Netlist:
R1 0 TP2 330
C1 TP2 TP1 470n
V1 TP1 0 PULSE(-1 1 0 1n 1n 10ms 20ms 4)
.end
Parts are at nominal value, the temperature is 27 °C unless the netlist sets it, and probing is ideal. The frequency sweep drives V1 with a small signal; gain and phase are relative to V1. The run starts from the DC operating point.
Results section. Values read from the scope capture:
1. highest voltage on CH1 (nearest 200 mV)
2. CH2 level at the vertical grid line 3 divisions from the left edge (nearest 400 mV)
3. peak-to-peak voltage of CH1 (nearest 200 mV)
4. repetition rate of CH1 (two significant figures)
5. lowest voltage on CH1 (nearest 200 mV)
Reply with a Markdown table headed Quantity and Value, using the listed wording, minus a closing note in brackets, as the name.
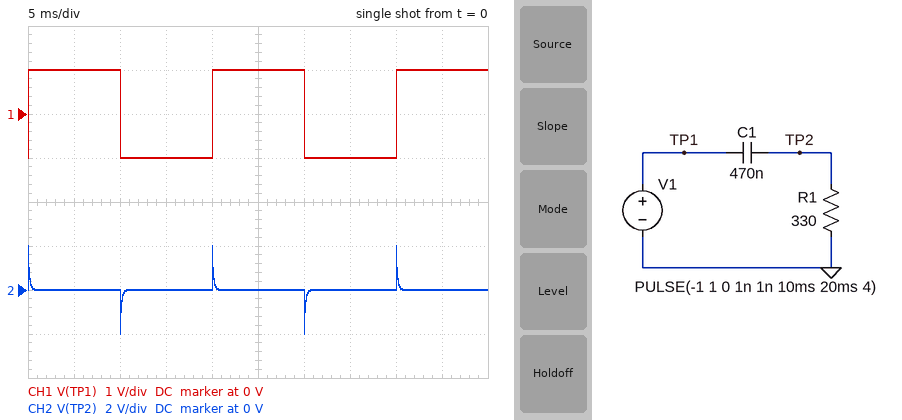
| Quantity | Value |
|---|---|
| highest voltage on CH1 | 1.0 V |
| CH2 level at the vertical grid line 3 divisions from the left edge | 0 V |
| peak-to-peak voltage of CH1 | 2.0 V |
| repetition rate of CH1 | 50 Hz |
| lowest voltage on CH1 | -1.0 V |
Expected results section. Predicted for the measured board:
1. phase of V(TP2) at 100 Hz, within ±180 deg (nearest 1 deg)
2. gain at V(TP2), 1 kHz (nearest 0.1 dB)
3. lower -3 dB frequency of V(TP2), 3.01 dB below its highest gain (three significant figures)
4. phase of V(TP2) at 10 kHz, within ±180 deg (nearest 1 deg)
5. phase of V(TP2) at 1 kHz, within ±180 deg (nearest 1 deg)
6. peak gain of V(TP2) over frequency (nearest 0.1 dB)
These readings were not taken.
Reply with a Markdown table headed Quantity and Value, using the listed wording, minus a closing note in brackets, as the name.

| Quantity | Value |
|---|---|
| phase of V(TP2) at 100 Hz, within ±180 deg | 84 deg |
| gain at V(TP2), 1 kHz | -3.1 dB |
| lower -3 dB frequency of V(TP2), 3.01 dB below its highest gain | 1.03 kHz |
| phase of V(TP2) at 10 kHz, within ±180 deg | 6 deg |
| phase of V(TP2) at 1 kHz, within ±180 deg | 46 deg |
| peak gain of V(TP2) over frequency | 0 dB |
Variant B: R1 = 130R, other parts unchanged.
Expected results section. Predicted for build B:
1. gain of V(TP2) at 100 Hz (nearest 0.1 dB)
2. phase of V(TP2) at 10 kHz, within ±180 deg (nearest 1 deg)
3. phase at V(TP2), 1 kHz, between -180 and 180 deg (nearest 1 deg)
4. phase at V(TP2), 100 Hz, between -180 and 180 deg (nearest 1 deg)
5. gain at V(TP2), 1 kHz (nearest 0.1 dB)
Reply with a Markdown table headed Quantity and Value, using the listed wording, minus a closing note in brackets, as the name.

| Quantity | Value |
|---|---|
| gain of V(TP2) at 100 Hz | -28.3 dB |
| phase of V(TP2) at 10 kHz, within ±180 deg | 15 deg |
| phase at V(TP2), 1 kHz, between -180 and 180 deg | 69 deg |
| phase at V(TP2), 100 Hz, between -180 and 180 deg | 88 deg |
| gain at V(TP2), 1 kHz | -8.9 dB |
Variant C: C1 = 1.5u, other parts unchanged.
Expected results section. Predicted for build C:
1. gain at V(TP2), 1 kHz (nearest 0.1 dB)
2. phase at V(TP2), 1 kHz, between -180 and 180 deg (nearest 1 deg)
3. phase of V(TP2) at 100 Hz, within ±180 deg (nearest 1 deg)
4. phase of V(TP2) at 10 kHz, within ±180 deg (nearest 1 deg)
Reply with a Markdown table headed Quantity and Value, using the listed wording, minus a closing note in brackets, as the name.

| Quantity | Value |
|---|---|
| gain at V(TP2), 1 kHz | -0.4 dB |
| phase at V(TP2), 1 kHz, between -180 and 180 deg | 18 deg |
| phase of V(TP2) at 100 Hz, within ±180 deg | 73 deg |
| phase of V(TP2) at 10 kHz, within ±180 deg | 2 deg |
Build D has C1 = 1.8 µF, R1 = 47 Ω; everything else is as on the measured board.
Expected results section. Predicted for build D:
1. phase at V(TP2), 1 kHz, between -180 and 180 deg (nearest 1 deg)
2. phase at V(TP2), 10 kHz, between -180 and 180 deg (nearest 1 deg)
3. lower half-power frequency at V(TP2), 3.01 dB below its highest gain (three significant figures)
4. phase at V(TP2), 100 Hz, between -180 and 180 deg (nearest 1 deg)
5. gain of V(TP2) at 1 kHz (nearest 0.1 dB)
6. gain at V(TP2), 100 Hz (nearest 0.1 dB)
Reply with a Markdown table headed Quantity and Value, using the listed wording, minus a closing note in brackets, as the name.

| Quantity | Value |
|---|---|
| phase at V(TP2), 1 kHz, between -180 and 180 deg | 62 deg |
| phase at V(TP2), 10 kHz, between -180 and 180 deg | 11 deg |
| lower half-power frequency at V(TP2), 3.01 dB below its highest gain | 1.88 kHz |
| phase at V(TP2), 100 Hz, between -180 and 180 deg | 87 deg |
| gain of V(TP2) at 1 kHz | -6.6 dB |
| gain at V(TP2), 100 Hz | -25.5 dB |
